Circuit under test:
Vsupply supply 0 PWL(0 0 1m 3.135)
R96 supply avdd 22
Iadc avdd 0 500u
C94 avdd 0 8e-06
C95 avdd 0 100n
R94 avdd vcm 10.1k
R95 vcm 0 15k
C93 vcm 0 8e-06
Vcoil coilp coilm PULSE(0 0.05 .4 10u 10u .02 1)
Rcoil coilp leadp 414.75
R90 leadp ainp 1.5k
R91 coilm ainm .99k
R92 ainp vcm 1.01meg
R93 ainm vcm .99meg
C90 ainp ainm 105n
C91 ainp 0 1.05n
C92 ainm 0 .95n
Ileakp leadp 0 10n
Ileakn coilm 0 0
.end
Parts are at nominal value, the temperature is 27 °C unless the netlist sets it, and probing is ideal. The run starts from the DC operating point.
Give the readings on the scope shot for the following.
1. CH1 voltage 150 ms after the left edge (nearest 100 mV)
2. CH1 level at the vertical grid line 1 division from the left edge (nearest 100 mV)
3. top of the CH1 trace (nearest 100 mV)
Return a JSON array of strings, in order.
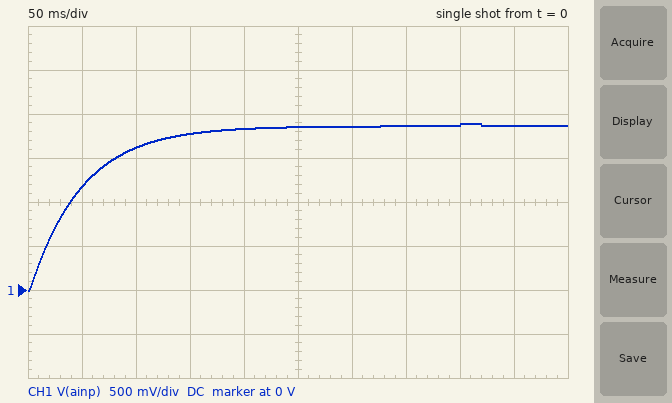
["1.8 V", "1.2 V", "1.9 V"]
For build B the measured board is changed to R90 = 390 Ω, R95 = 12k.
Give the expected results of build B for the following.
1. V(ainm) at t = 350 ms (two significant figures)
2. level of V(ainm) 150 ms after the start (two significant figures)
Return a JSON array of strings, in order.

["1.7 V", "1.6 V"]
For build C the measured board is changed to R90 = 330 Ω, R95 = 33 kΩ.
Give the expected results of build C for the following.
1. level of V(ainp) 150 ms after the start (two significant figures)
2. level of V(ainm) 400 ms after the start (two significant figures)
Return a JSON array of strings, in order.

["2.2 V", "2.4 V"]
